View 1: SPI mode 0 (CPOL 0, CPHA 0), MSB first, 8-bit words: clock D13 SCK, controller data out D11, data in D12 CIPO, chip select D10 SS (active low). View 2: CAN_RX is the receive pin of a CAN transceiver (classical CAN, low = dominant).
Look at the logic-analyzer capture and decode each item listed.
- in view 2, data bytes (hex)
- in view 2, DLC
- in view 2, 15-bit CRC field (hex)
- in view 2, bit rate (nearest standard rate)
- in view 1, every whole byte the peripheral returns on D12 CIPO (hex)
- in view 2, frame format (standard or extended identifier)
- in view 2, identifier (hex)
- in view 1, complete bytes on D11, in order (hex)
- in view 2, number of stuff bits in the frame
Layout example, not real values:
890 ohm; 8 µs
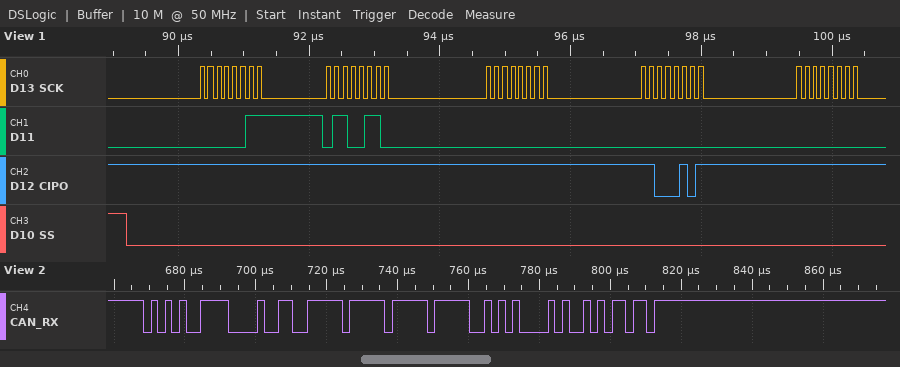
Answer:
CF FF FF 54; 4; 0x14AD; 500 kbit/s; FF FF FF C5 FF; standard; 0x54F; 03 66 00 00 00; 4
